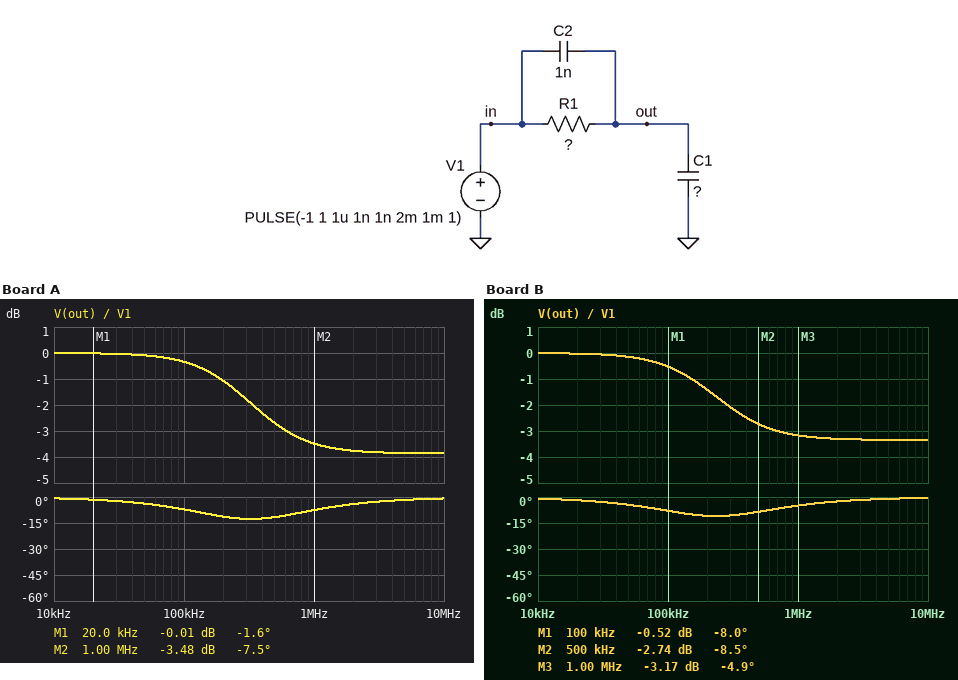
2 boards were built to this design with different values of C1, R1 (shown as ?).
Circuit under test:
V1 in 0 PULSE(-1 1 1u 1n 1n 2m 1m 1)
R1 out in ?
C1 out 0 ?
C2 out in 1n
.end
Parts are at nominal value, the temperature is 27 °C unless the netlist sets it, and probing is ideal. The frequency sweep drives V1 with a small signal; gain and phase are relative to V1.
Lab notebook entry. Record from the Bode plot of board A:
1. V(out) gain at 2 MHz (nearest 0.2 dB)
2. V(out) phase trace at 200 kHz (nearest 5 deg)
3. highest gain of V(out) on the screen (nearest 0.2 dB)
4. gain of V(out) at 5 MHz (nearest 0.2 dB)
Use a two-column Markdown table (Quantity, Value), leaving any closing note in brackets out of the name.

| Quantity | Value |
|---|---|
| V(out) gain at 2 MHz | -3.8 dB |
| V(out) phase trace at 200 kHz | -10 deg |
| highest gain of V(out) on the screen | 0 dB |
| gain of V(out) at 5 MHz | -3.8 dB |
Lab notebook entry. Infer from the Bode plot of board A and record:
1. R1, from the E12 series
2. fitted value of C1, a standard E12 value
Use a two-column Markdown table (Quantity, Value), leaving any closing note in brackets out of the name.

| Quantity | Value |
|---|---|
| R1, from the E12 series | 390 Ω |
| fitted value of C1, a standard E12 value | 560 pF |
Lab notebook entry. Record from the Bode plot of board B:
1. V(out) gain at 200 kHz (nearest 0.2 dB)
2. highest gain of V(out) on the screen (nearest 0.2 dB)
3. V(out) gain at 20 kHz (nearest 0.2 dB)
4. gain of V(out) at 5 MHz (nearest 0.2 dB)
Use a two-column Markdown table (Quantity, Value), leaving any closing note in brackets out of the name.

| Quantity | Value |
|---|---|
| V(out) gain at 200 kHz | -1.4 dB |
| highest gain of V(out) on the screen | 0 dB |
| V(out) gain at 20 kHz | 0 dB |
| gain of V(out) at 5 MHz | -3.4 dB |
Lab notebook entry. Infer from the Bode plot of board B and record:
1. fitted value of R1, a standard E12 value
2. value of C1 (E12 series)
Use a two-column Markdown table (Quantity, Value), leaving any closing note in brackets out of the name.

| Quantity | Value |
|---|---|
| fitted value of R1, a standard E12 value | 560 Ω |
| value of C1 | 470 pF |
